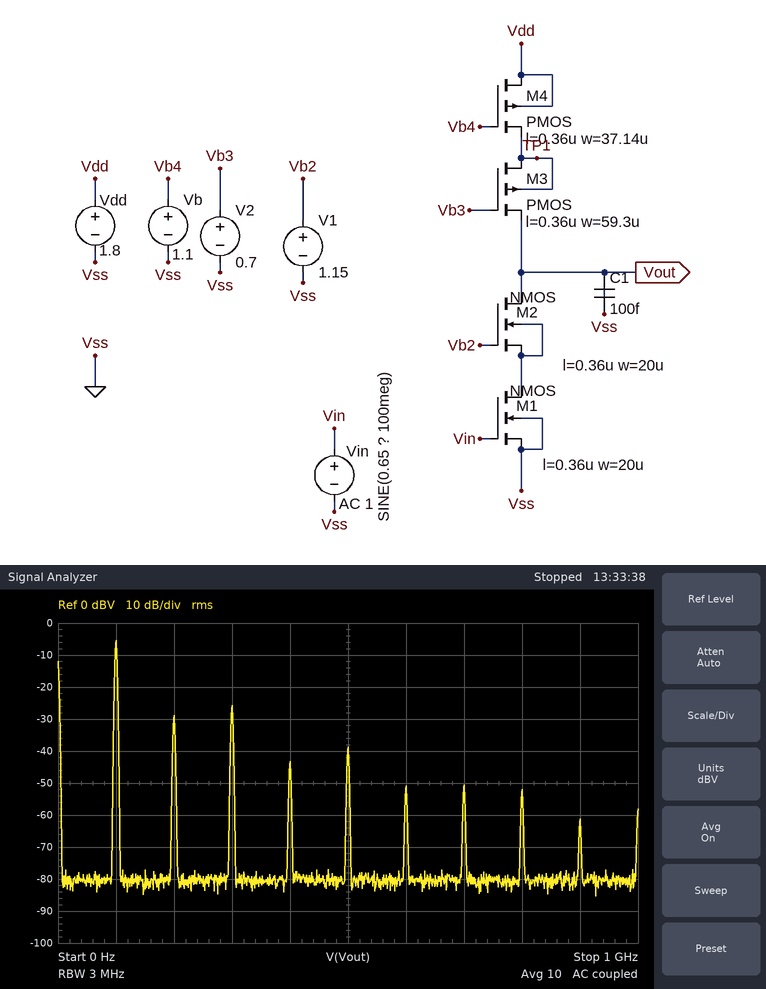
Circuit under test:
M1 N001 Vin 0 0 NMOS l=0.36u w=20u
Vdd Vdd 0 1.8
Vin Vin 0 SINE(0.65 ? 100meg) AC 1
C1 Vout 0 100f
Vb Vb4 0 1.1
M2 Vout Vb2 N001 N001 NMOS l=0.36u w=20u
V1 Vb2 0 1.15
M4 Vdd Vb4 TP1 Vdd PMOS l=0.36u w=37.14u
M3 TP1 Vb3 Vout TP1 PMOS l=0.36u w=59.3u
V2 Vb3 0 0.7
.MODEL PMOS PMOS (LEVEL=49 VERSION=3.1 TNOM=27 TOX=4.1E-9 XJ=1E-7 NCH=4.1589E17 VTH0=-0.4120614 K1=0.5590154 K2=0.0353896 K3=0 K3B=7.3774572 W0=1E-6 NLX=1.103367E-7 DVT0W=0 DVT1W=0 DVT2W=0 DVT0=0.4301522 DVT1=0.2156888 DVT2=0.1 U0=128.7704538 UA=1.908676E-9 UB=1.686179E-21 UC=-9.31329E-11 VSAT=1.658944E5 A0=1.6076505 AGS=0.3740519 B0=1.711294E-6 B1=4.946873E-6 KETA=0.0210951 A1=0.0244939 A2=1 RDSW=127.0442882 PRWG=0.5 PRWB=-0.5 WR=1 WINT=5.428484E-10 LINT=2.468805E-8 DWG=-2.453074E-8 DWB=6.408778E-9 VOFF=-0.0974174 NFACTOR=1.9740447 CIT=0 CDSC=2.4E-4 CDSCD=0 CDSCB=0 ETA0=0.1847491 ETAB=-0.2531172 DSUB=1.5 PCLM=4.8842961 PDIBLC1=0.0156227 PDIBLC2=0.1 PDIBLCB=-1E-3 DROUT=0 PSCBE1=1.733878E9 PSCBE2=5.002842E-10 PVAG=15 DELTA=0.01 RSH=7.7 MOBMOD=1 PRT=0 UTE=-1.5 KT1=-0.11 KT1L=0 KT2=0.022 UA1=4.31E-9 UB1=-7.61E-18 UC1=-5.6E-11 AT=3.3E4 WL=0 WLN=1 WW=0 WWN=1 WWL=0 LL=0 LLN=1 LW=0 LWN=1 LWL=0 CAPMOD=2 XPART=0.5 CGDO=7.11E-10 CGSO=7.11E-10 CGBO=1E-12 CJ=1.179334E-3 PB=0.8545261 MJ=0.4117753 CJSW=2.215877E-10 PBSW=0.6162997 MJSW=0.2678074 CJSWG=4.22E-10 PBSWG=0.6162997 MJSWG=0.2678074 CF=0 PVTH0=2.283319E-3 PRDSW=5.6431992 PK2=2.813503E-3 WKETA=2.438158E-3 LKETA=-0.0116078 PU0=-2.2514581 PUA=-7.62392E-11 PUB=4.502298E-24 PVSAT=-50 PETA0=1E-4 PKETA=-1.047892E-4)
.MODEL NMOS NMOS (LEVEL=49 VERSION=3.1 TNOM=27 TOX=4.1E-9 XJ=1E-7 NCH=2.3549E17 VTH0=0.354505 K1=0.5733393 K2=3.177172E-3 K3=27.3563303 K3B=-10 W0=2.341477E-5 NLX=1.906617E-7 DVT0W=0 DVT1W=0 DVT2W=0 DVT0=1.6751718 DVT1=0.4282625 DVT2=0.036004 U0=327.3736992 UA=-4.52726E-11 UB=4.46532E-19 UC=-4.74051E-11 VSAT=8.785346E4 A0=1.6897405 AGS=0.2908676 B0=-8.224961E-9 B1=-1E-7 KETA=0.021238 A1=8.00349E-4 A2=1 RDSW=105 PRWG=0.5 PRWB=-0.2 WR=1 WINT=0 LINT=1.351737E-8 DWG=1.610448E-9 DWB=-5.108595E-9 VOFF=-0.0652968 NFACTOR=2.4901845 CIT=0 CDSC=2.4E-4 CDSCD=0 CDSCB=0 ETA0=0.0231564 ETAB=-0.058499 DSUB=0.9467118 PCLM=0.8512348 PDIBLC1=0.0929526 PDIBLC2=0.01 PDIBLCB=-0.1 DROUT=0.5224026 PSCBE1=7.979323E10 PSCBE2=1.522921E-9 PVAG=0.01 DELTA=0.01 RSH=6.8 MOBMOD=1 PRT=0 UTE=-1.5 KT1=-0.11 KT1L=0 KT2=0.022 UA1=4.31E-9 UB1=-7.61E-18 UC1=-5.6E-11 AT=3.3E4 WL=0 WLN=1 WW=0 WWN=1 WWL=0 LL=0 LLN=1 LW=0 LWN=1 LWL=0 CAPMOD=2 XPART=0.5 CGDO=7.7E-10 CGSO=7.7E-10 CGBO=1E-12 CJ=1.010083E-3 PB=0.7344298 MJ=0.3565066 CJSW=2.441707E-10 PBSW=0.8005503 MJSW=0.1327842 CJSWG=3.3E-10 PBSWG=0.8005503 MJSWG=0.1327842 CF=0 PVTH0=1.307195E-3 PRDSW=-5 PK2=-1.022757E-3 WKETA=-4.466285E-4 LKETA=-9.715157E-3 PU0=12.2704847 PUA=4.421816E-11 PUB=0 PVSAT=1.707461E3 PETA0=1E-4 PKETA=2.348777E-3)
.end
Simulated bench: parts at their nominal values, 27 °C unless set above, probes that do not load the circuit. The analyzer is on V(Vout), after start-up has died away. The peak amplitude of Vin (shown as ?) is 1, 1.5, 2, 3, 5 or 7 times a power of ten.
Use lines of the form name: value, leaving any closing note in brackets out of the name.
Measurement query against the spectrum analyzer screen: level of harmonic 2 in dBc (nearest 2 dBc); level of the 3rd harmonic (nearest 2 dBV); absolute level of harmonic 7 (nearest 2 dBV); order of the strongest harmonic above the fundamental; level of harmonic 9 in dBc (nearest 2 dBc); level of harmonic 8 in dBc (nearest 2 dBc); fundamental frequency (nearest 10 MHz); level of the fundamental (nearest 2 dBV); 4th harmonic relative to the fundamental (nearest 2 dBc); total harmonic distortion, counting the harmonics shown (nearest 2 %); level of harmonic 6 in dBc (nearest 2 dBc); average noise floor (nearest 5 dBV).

level of harmonic 2 in dBc: -24 dBc
level of the 3rd harmonic: -26 dBV
absolute level of harmonic 7: -50 dBV
order of the strongest harmonic above the fundamental: 3
level of harmonic 9 in dBc: -56 dBc
level of harmonic 8 in dBc: -46 dBc
fundamental frequency: 100 MHz
level of the fundamental: -6 dBV
4th harmonic relative to the fundamental: -38 dBc
total harmonic distortion, counting the harmonics shown: 12 %
level of harmonic 6 in dBc: -46 dBc
average noise floor: -80 dBV
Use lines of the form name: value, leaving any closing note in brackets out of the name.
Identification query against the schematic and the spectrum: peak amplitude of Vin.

peak amplitude of Vin: 50 mV
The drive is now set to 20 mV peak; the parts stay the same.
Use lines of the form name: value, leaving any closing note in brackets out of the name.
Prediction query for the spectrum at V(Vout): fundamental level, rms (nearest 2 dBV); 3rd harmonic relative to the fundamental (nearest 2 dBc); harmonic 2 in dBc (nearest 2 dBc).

fundamental level, rms: -10 dBV
3rd harmonic relative to the fundamental: -32 dBc
harmonic 2 in dBc: -28 dBc
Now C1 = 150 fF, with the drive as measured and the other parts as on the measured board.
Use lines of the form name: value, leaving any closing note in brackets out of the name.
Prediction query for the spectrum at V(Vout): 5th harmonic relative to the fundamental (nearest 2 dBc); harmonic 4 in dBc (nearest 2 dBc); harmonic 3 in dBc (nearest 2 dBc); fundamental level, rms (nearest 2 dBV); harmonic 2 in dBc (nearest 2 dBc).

5th harmonic relative to the fundamental: -54 dBc
harmonic 4 in dBc: -36 dBc
harmonic 3 in dBc: -24 dBc
fundamental level, rms: -6 dBV
harmonic 2 in dBc: -22 dBc
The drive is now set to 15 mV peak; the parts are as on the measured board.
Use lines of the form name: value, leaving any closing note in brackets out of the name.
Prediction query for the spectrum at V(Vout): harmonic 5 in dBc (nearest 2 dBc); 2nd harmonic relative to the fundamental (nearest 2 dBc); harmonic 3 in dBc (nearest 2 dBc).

harmonic 5 in dBc: -50 dBc
2nd harmonic relative to the fundamental: -38 dBc
harmonic 3 in dBc: -38 dBc
